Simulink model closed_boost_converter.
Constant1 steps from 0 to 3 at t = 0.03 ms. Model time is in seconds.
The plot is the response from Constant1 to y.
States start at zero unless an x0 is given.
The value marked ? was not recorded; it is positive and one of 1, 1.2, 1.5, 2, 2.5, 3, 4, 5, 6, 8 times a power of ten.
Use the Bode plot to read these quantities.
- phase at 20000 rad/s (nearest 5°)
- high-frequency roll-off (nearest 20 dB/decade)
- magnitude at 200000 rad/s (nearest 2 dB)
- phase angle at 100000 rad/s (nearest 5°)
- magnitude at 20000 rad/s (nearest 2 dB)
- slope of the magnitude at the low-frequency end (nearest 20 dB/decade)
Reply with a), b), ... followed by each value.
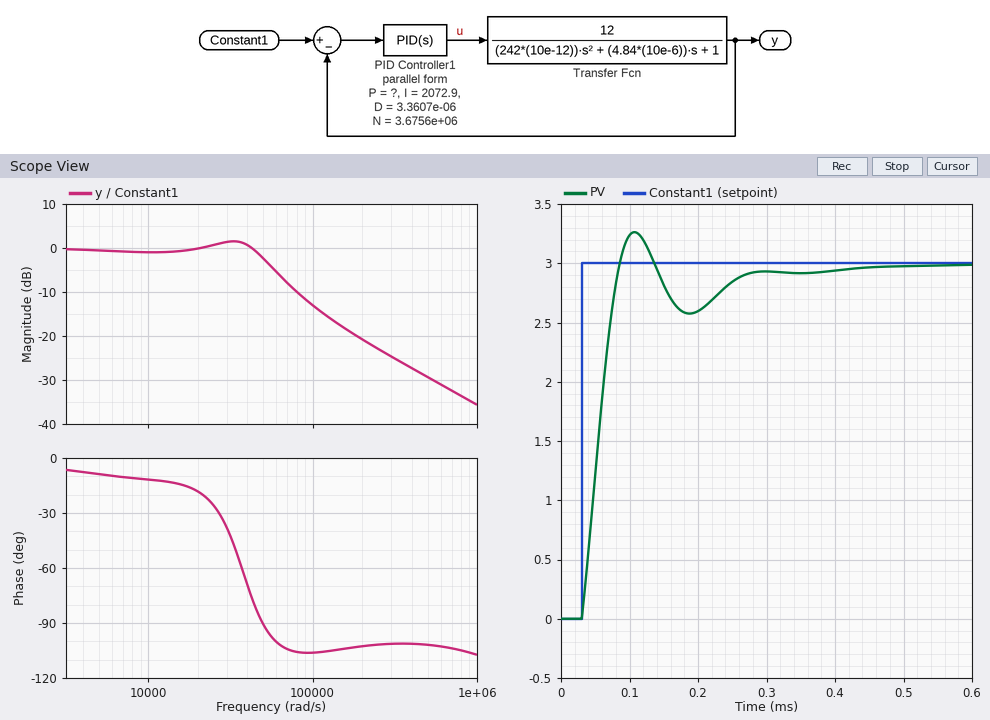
a) -20°
b) -20 dB/decade
c) -20 dB
d) -105°
e) 0 dB
f) 0 dB/decade
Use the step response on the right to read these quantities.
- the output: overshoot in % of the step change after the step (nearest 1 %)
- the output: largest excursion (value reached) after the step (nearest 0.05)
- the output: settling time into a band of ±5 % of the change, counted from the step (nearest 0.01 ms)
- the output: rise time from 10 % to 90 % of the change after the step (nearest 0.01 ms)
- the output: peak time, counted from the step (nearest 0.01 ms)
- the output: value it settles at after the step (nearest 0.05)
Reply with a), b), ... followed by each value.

a) 9 %
b) 3.25
c) 0.22 ms
d) 0.04 ms
e) 0.08 ms
f) 3.00
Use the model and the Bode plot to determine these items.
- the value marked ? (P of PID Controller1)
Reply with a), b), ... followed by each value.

a) 0.25
